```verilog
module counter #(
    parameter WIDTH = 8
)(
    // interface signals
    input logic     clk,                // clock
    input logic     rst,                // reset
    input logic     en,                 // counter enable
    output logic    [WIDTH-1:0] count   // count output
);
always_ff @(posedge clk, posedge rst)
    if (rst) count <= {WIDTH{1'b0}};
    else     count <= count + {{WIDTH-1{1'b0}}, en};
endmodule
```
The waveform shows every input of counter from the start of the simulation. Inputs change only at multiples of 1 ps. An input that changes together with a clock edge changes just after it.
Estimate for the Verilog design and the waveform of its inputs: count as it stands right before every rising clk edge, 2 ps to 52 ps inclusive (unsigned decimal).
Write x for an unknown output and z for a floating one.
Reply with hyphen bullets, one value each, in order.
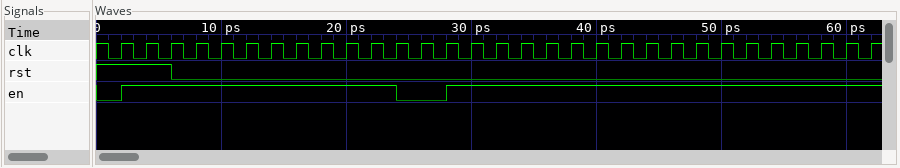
- 0, 0, 0, 0, 1, 2, 3, 4, 5, 6, 7, 8, 9, 9, 9, 10, 11, 12, 13, 14, 15, 16, 17, 18, 19, 20
